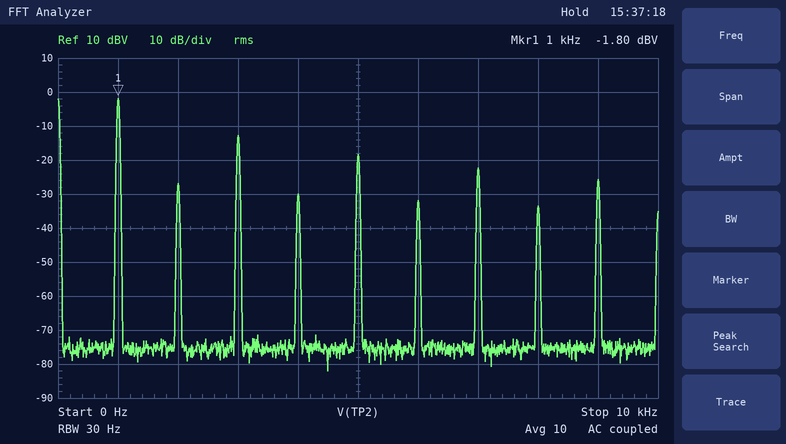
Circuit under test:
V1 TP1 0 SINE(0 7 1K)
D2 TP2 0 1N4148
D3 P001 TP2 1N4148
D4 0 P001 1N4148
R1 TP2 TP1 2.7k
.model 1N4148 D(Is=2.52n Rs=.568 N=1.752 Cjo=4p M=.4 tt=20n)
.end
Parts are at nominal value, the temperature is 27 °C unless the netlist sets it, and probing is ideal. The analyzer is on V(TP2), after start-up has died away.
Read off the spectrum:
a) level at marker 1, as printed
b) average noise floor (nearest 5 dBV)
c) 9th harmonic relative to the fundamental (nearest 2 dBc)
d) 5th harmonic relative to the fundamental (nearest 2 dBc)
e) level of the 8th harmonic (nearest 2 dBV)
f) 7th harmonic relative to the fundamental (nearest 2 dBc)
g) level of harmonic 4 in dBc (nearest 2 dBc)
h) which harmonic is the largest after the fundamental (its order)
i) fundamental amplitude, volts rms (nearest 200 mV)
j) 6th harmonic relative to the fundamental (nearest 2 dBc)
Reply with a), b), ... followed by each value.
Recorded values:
a) -1.80 dBV
b) -75 dBV
c) -24 dBc
d) -16 dBc
e) -34 dBV
f) -20 dBc
g) -28 dBc
h) 3
i) 800 mV
j) -30 dBc
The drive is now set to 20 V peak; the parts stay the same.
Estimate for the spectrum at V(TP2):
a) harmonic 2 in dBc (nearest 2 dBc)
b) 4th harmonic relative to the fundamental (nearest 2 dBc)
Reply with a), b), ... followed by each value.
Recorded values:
a) -30 dBc
b) -34 dBc
